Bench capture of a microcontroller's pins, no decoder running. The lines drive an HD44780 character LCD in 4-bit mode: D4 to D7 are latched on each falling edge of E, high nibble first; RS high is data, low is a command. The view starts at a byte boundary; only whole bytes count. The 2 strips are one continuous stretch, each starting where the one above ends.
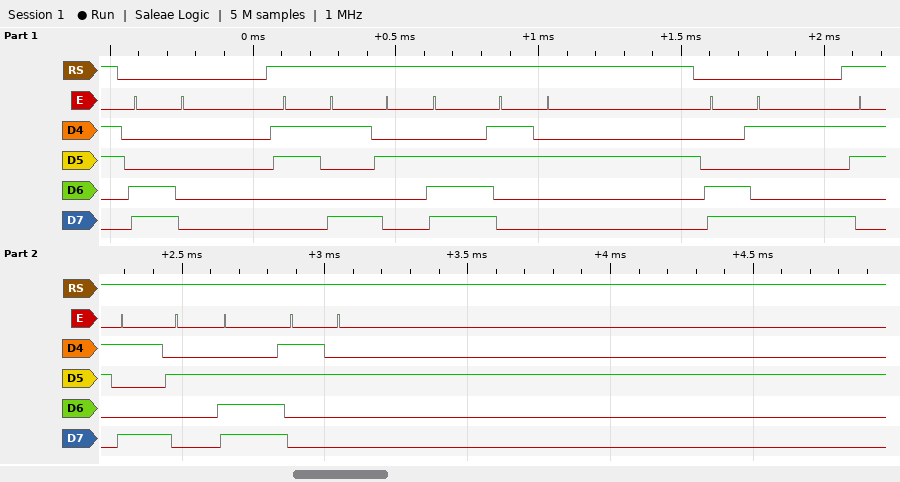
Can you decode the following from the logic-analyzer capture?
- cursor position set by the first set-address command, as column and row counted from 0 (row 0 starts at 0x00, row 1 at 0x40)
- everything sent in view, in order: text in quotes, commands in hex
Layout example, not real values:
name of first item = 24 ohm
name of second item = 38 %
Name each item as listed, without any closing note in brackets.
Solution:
cursor position set by the first set-address command, as column and row counted from 0 = column 0, row 1
everything sent in view, in order: text in quotes, commands in hex = 0xC0 "9.2" 0xC9 "9.2"
